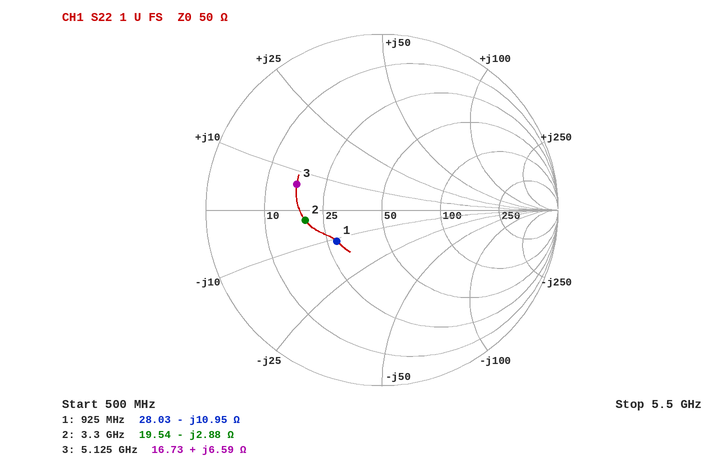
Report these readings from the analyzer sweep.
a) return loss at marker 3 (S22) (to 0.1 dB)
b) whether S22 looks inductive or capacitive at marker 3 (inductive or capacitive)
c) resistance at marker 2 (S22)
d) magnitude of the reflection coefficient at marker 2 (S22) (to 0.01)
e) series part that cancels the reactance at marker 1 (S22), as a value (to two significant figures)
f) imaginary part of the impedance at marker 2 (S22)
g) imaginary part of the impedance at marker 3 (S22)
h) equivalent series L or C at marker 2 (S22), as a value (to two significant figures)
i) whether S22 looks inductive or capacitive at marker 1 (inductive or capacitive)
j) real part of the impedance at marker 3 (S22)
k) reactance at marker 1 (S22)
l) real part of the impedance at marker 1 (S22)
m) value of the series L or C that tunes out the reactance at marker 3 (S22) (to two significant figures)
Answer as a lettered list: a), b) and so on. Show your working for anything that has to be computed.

a) 5.9 dB
b) inductive
c) 19.54 Ω
d) 0.44
e) L = 10.95 Ω/(2π × 925 MHz) ≈ 1.9 nH
f) -2.88 Ω
g) +6.59 Ω
h) C = 1/(2π × 3.3 GHz × 2.88 Ω) ≈ 17 pF
i) capacitive
j) 16.73 Ω
k) -10.95 Ω
l) 28.03 Ω
m) C = 1/(2π × 5.125 GHz × 6.59 Ω) ≈ 4.7 pF
